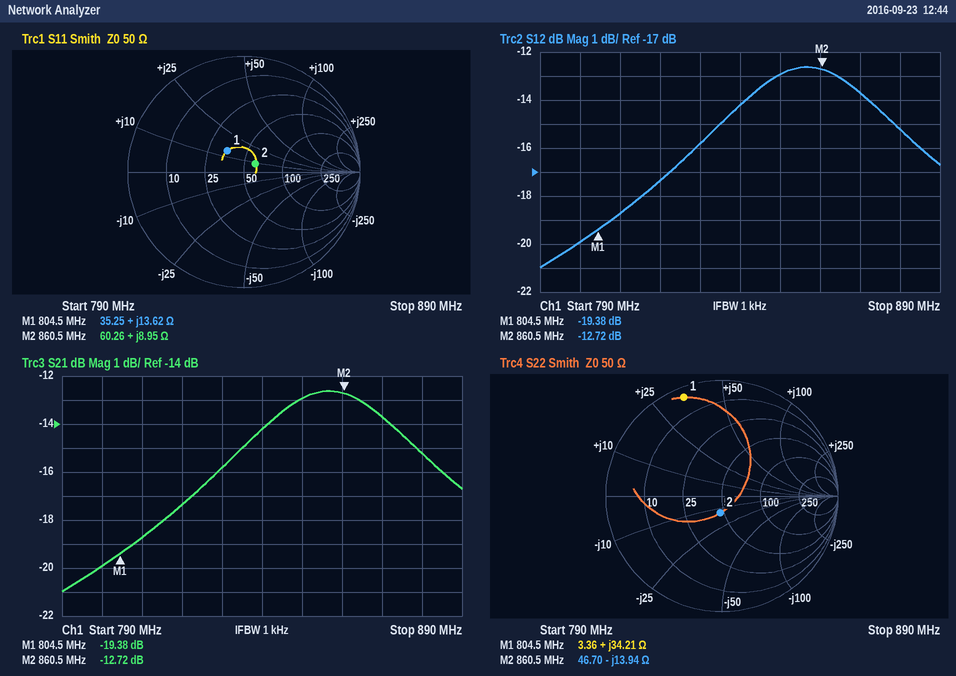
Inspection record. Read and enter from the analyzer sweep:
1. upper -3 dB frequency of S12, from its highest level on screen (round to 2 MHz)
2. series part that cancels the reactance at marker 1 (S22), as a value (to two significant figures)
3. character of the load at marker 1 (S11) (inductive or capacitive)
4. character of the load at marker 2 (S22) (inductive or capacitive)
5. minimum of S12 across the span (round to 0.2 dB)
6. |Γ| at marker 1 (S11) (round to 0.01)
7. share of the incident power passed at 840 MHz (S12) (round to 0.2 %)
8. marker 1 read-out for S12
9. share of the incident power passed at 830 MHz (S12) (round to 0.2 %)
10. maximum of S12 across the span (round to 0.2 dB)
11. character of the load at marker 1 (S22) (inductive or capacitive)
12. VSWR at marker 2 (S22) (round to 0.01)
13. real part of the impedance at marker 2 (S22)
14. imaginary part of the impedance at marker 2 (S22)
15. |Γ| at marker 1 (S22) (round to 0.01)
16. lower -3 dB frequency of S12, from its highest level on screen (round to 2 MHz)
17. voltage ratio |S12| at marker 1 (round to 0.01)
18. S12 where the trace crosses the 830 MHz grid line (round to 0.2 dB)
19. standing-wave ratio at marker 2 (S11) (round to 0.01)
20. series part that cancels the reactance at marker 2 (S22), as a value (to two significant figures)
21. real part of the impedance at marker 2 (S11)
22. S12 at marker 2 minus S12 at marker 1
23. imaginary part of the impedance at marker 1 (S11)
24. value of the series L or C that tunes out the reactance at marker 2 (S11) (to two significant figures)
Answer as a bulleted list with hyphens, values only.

- 882 MHz
- 5.8 pF
- inductive
- capacitive
- -21.0 dB
- 0.23
- 3.8 %
- -19.38 dB
- 2.6 %
- -12.6 dB
- inductive
- 1.34
- 46.70 Ω
- -13.94 Ω
- 0.91
- 832 MHz
- 0.11
- -15.8 dB
- 1.28
- 2.6 nH
- 60.26 Ω
- 6.66 dB
- +13.62 Ω
- 21 pF
